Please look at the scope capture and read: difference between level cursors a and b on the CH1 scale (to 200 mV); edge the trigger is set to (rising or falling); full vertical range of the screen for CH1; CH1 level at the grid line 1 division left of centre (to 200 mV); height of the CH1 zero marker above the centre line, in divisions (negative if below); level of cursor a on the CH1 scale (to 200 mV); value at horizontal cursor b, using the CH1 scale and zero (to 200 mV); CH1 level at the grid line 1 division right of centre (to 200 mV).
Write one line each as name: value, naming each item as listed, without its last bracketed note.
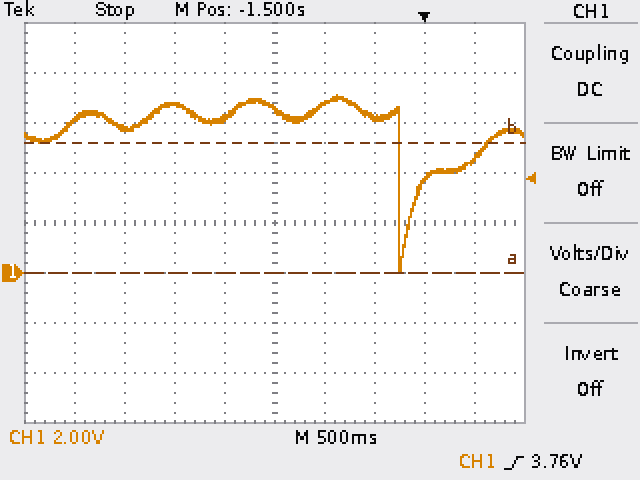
difference between level cursors a and b on the CH1 scale: 5.2 V
edge the trigger is set to: rising
full vertical range of the screen for CH1: 16 V
CH1 level at the grid line 1 division left of centre: 6.2 V
height of the CH1 zero marker above the centre line, in divisions: -1.0 div
level of cursor a on the CH1 scale: 0.0 V
value at horizontal cursor b, using the CH1 scale and zero: 5.2 V
CH1 level at the grid line 1 division right of centre: 6.8 V
